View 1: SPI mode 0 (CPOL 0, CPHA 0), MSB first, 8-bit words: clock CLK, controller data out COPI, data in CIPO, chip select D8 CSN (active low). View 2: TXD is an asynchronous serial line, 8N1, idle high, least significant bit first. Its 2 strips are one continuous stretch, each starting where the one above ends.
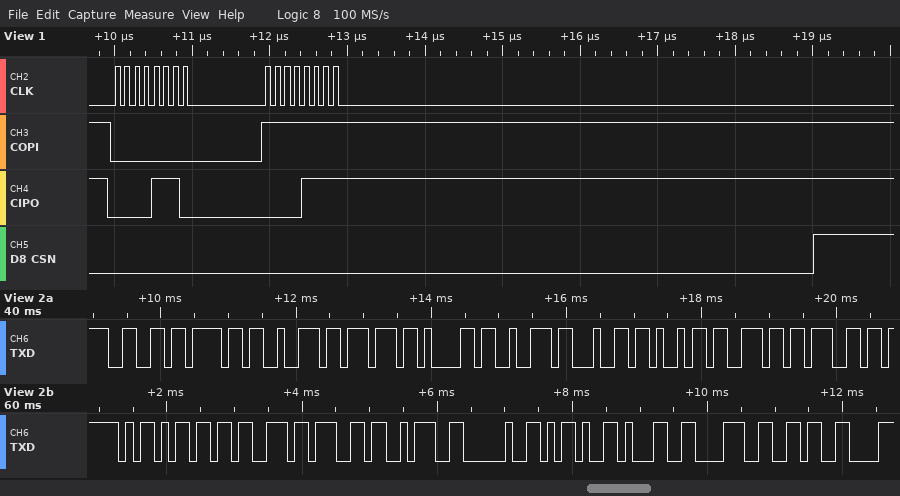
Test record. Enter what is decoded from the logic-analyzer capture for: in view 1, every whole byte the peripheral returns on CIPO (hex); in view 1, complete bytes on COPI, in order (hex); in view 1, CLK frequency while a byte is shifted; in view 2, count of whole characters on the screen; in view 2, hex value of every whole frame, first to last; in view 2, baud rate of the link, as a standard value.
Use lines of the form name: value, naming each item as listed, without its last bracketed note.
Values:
in view 1, every whole byte the peripheral returns on CIPO: 0E 0F
in view 1, complete bytes on COPI, in order: 00 FF
in view 1, CLK frequency while a byte is shifted: 8 MHz
in view 2, count of whole characters on the screen: 20
in view 2, hex value of every whole frame, first to last: 0x66 0x6F 0x72 0x77 0x61 0x72 0x64 0x69 0x6E 0x67 0x5F 0x6D 0x73 0x67 0x3A 0x20 0x2D 0x31 0x38 0x36
in view 2, baud rate of the link, as a standard value: 9600 baud
